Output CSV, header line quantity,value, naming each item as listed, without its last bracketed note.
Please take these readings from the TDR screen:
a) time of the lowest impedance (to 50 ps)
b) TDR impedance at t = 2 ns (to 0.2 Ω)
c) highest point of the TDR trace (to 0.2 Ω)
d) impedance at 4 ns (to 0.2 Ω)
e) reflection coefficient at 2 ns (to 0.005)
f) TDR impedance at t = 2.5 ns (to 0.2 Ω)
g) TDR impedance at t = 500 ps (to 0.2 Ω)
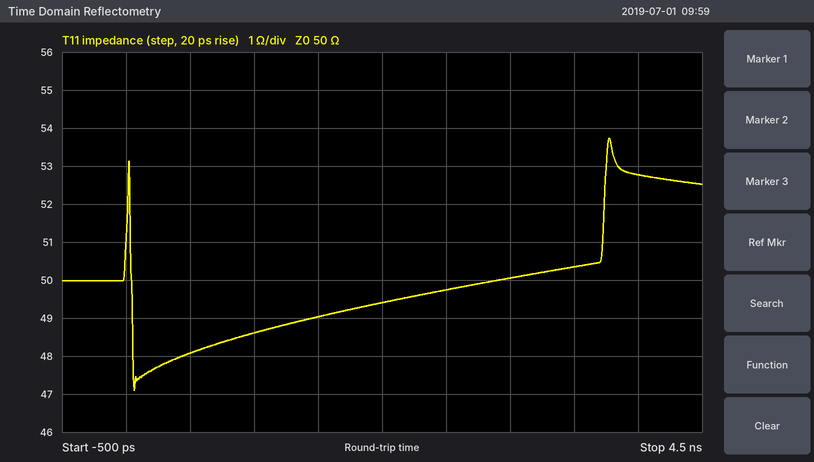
quantity,value
time of the lowest impedance,50 ps
TDR impedance at t = 2 ns,49.4 Ω
highest point of the TDR trace,53.8 Ω
impedance at 4 ns,52.8 Ω
reflection coefficient at 2 ns,-0.005
TDR impedance at t = 2.5 ns,49.8 Ω
TDR impedance at t = 500 ps,48.0 Ω
